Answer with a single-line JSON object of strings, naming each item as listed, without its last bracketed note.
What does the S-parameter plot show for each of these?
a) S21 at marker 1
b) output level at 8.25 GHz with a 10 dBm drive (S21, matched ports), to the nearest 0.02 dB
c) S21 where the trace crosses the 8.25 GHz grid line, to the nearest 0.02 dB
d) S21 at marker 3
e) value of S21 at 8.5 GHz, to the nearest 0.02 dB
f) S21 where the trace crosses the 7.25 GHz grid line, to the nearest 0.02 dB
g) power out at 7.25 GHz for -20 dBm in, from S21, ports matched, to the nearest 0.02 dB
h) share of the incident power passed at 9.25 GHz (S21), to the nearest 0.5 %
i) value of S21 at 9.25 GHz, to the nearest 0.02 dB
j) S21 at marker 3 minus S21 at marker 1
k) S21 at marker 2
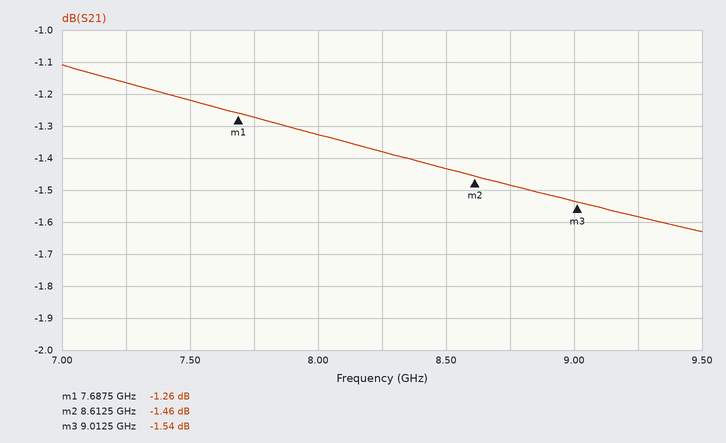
{"S21 at marker 1": "-1.26 dB", "output level at 8.25 GHz with a 10 dBm drive (S21, matched ports), to the nearest 0.02 dB": "8.62 dBm", "S21 where the trace crosses the 8.25 GHz grid line, to the nearest 0.02 dB": "-1.38 dB", "S21 at marker 3": "-1.54 dB", "value of S21 at 8.5 GHz, to the nearest 0.02 dB": "-1.44 dB", "S21 where the trace crosses the 7.25 GHz grid line, to the nearest 0.02 dB": "-1.16 dB", "power out at 7.25 GHz for -20 dBm in, from S21, ports matched, to the nearest 0.02 dB": "-21.16 dBm", "share of the incident power passed at 9.25 GHz (S21), to the nearest 0.5 %": "69.5 %", "value of S21 at 9.25 GHz, to the nearest 0.02 dB": "-1.58 dB", "S21 at marker 3 minus S21 at marker 1": "-0.28 dB", "S21 at marker 2": "-1.46 dB"}
